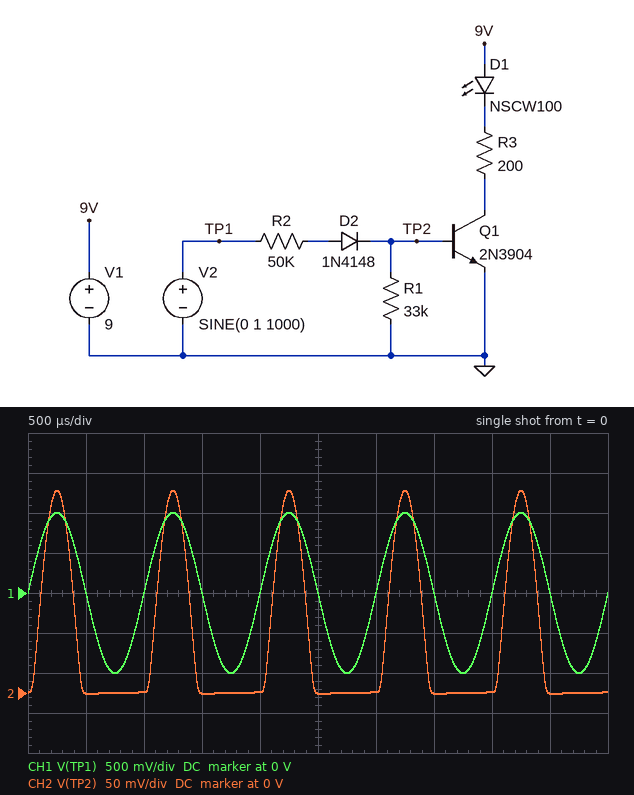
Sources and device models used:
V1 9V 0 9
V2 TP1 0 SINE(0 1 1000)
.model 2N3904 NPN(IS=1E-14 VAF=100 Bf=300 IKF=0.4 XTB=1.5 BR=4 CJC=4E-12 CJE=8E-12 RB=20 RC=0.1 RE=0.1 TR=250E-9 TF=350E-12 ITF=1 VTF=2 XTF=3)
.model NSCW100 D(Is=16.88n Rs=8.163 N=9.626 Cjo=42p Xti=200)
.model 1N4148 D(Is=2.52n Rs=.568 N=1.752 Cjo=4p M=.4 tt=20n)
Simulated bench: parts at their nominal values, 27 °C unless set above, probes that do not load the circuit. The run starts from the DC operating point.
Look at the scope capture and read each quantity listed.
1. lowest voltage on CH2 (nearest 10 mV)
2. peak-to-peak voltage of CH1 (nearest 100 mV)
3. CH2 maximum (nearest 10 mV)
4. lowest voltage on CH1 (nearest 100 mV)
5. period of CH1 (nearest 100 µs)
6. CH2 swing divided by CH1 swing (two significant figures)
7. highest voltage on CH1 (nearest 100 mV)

0 V
2.0 V
250 mV
-1.0 V
1.0 ms
0.13
1.0 V
